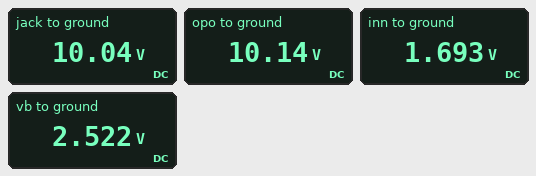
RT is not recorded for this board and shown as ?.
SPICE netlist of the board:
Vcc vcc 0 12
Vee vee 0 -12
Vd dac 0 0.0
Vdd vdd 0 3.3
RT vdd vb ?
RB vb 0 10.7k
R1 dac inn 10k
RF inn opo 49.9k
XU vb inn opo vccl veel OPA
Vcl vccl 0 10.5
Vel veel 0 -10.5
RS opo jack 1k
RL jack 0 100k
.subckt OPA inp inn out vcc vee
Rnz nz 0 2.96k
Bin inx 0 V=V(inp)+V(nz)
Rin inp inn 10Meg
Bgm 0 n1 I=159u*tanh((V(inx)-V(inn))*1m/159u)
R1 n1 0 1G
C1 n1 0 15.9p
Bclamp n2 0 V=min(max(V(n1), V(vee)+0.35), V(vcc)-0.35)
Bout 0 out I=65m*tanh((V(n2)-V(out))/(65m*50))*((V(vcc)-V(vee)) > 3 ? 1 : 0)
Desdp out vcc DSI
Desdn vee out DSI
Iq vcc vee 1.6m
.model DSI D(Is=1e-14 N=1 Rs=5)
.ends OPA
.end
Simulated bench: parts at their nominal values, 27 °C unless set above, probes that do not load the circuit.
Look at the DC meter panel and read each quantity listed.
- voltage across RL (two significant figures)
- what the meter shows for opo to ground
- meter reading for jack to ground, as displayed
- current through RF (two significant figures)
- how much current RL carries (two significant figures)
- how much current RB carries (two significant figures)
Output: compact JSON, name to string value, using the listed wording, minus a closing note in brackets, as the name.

{"voltage across RL": "10 V", "what the meter shows for opo to ground": "10.14 V", "meter reading for jack to ground, as displayed": "10.04 V", "current through RF": "170 µA", "how much current RL carries": "100 µA", "how much current RB carries": "240 µA"}
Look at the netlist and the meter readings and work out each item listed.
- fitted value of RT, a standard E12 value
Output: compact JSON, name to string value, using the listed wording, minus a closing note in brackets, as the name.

{"fitted value of RT, a standard E12 value": "3.3 kΩ"}
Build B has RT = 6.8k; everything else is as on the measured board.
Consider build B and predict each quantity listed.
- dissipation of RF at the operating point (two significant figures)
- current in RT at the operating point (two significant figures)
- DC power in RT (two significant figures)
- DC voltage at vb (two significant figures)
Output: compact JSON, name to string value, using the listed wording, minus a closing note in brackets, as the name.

{"dissipation of RF at the operating point": "1.4 mW", "current in RT at the operating point": "190 µA", "DC power in RT": "240 µW", "DC voltage at vb": "2.0 V"}
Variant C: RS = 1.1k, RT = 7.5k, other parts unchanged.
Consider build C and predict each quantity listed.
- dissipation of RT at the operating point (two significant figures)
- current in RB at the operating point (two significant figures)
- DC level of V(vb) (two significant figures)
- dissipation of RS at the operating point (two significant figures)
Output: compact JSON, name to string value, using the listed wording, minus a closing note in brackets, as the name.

{"dissipation of RT at the operating point": "250 µW", "current in RB at the operating point": "180 µA", "DC level of V(vb)": "1.9 V", "dissipation of RS at the operating point": "11 µW"}
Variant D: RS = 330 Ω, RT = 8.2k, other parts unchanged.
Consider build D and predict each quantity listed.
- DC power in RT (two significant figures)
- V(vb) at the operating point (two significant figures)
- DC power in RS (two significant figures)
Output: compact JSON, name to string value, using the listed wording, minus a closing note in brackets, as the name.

{"DC power in RT": "250 µW", "V(vb) at the operating point": "1.9 V", "DC power in RS": "3.4 µW"}
